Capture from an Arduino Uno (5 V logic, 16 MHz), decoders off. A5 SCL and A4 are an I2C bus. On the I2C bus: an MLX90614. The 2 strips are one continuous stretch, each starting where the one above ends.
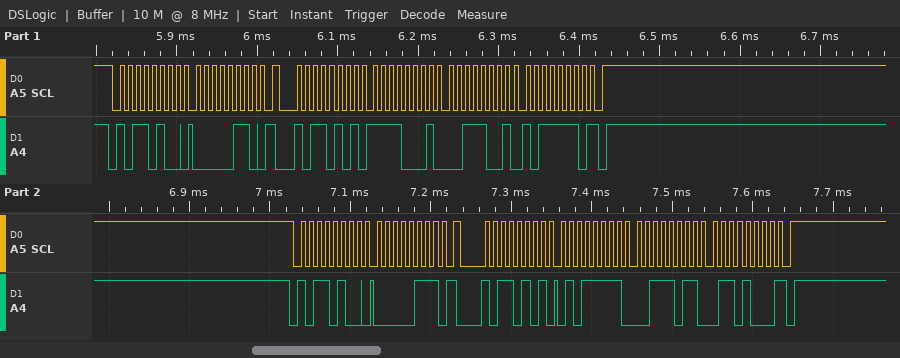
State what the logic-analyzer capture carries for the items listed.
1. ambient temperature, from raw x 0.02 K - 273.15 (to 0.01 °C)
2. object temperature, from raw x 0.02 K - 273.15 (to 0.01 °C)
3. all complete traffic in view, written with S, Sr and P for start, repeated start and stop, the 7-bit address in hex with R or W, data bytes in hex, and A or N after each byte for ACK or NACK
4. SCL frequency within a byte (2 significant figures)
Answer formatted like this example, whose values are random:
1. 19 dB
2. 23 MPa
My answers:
1. 23.51 °C
2. 30.83 °C
3. S 5AW A 06 A Sr 5AR A F1 A 39 A BE N P S 5AW A 07 A Sr 5AR A 5F A 3B A 68 N P
4. 100 kHz
